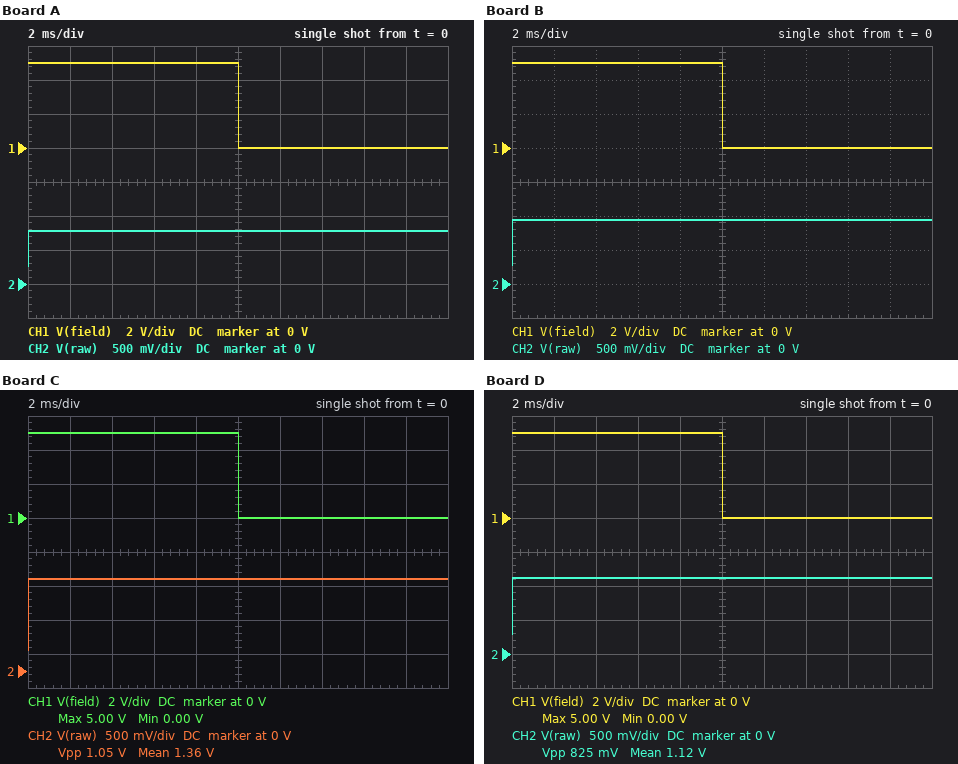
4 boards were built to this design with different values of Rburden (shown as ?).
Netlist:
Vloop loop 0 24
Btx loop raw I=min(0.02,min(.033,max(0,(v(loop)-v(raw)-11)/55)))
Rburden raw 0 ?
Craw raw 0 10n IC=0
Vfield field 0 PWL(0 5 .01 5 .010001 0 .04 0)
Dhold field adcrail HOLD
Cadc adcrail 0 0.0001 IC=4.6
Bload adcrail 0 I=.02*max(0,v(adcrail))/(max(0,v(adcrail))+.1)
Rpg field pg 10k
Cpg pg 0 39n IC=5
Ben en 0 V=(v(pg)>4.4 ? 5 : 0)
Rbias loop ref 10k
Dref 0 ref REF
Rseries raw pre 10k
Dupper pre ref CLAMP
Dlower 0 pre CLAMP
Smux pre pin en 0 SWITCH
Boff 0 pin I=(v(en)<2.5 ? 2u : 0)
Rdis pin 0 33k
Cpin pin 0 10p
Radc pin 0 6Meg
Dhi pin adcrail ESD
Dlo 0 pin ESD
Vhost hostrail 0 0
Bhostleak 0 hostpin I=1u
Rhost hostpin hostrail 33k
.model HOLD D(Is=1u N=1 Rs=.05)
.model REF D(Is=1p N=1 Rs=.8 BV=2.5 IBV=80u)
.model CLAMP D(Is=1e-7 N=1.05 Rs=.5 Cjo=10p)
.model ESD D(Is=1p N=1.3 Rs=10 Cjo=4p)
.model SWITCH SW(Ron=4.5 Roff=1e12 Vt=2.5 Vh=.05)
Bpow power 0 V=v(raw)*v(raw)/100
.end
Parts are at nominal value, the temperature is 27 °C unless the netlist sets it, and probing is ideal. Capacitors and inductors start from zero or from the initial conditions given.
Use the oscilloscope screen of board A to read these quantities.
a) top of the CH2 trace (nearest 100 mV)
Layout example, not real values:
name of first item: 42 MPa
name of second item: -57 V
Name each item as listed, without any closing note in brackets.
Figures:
top of the CH2 trace: 800 mV
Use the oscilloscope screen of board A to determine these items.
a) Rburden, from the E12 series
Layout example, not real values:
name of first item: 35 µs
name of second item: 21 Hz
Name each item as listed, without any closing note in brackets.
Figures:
Rburden, from the E12 series: 39 Ω
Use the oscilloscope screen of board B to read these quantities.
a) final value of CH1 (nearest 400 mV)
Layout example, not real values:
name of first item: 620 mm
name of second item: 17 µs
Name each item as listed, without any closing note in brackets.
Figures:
final value of CH1: 0 V
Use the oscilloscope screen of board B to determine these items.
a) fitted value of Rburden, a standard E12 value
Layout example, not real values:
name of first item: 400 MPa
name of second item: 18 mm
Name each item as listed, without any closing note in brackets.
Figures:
fitted value of Rburden, a standard E12 value: 47 Ω
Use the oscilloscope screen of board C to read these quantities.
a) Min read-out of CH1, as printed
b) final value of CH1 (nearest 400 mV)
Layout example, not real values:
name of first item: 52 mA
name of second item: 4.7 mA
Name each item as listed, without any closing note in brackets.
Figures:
Min read-out of CH1, as printed: 0.00 V
final value of CH1: 0 V
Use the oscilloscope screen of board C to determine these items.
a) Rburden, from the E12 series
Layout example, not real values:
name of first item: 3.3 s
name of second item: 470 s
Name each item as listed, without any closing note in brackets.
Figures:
Rburden, from the E12 series: 68 Ω
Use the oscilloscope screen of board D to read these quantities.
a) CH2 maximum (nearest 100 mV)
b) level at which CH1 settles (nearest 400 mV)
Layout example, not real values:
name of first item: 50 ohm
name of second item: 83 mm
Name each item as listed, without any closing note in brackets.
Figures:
CH2 maximum: 1.1 V
level at which CH1 settles: 0 V
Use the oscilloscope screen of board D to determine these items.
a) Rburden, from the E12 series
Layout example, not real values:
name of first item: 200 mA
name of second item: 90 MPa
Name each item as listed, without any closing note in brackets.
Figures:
Rburden, from the E12 series: 56 Ω
